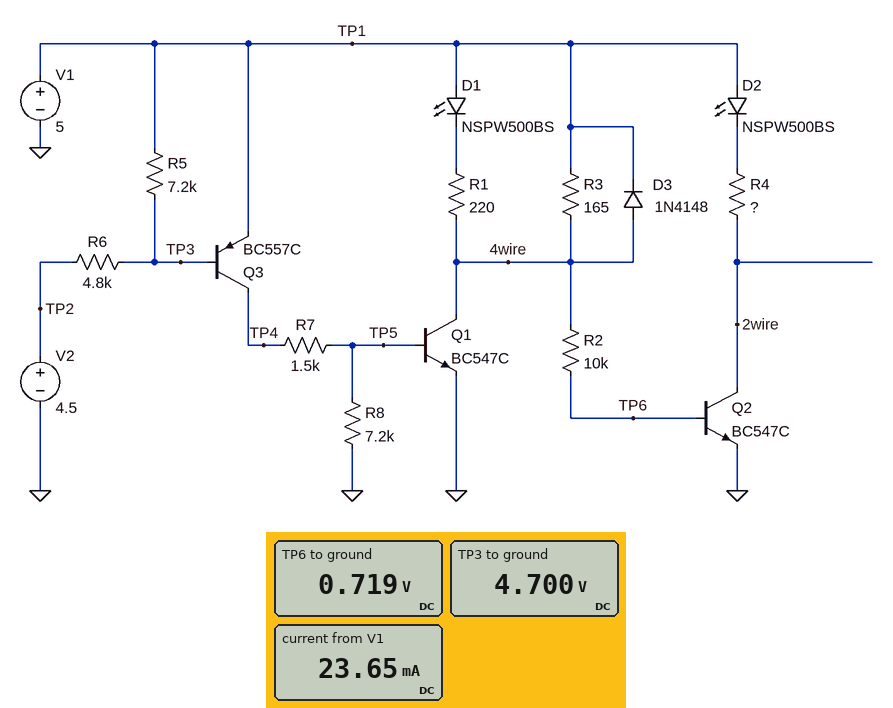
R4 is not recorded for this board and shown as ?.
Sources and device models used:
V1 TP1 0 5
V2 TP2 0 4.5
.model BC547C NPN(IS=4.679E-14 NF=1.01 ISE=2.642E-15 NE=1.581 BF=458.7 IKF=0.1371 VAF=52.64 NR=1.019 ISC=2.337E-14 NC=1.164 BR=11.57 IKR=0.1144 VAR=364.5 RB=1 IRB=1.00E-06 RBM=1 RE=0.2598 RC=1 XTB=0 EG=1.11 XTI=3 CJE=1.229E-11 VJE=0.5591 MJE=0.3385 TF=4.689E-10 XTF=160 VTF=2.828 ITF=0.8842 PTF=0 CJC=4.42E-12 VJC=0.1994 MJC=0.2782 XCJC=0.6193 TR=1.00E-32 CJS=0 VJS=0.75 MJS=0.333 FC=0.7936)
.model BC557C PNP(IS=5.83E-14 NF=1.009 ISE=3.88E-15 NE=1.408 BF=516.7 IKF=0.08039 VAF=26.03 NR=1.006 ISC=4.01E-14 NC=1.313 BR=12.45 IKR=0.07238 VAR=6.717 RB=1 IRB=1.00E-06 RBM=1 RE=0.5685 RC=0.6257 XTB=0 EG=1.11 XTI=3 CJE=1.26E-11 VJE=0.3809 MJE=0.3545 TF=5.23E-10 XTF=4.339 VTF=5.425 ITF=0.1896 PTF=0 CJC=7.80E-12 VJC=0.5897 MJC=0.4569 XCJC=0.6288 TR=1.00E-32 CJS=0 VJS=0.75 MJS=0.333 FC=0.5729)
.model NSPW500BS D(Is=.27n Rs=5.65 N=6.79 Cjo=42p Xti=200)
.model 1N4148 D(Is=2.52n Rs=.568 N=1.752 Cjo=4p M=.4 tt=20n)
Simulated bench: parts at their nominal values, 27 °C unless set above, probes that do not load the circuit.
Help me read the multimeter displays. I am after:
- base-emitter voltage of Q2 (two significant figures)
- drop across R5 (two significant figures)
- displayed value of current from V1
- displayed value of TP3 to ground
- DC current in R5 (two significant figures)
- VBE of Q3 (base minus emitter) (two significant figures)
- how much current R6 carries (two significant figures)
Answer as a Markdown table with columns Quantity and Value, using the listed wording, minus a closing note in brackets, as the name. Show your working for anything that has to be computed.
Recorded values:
| Quantity | Value |
|---|---|
| base-emitter voltage of Q2 | 719 mV = 720 mV |
| drop across R5 | 5 V - 4.7 V = 300 mV |
| displayed value of current from V1 | 23.65 mA |
| displayed value of TP3 to ground | 4.700 V |
| DC current in R5 | (5 V - 4.7 V) / 7.2 kΩ = 42 µA |
| VBE of Q3 (base minus emitter) | 4.7 V - 5 V = -300 mV |
| how much current R6 carries | (4.7 V - 4.5 V) / 4.8 kΩ = 42 µA |
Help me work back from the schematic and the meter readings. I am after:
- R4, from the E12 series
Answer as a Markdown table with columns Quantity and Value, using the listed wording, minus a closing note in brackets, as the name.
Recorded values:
| Quantity | Value |
|---|---|
| R4, from the E12 series | 68 Ω |
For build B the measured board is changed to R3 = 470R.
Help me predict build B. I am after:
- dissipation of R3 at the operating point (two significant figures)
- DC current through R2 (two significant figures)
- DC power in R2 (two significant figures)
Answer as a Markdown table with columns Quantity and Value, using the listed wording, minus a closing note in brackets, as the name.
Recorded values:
| Quantity | Value |
|---|---|
| dissipation of R3 at the operating point | 79 µW |
| DC current through R2 | 410 µA |
| DC power in R2 | 1.7 mW |
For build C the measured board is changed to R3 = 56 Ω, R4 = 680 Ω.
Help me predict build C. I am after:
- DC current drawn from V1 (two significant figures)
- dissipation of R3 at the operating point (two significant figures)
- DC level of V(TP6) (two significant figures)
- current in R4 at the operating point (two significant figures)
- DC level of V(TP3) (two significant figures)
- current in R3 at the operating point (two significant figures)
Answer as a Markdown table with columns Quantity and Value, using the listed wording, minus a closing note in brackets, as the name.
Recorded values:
| Quantity | Value |
|---|---|
| DC current drawn from V1 | 3.6 mA |
| dissipation of R3 at the operating point | 10 µW |
| DC level of V(TP6) | 680 mV |
| current in R4 at the operating point | 3.1 mA |
| DC level of V(TP3) | 4.7 V |
| current in R3 at the operating point | 430 µA |
